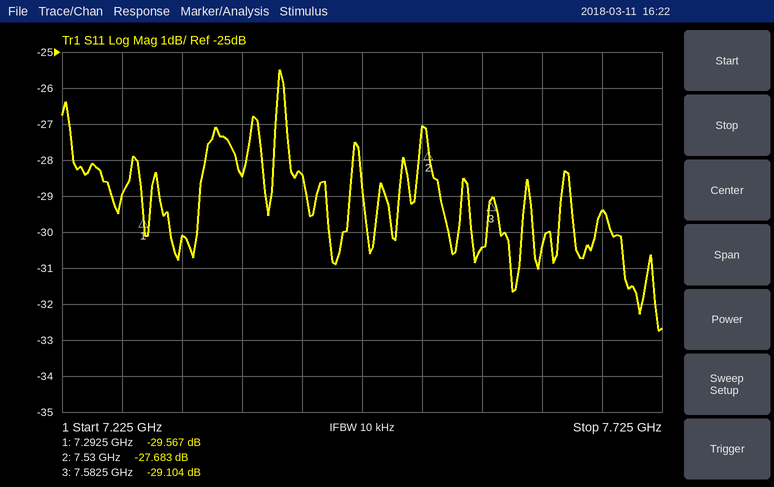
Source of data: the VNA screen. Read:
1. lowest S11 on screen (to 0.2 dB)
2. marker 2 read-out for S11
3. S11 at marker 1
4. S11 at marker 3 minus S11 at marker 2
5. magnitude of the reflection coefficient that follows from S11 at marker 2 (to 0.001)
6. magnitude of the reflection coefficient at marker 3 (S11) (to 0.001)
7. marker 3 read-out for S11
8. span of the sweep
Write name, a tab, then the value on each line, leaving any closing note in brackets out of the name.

lowest S11 on screen	-32.8 dB
marker 2 read-out for S11	-27.683 dB
S11 at marker 1	-29.567 dB
S11 at marker 3 minus S11 at marker 2	-1.421 dB
magnitude of the reflection coefficient that follows from S11 at marker 2	0.041
magnitude of the reflection coefficient at marker 3 (S11)	0.035
marker 3 read-out for S11	-29.104 dB
span of the sweep	500 MHz
